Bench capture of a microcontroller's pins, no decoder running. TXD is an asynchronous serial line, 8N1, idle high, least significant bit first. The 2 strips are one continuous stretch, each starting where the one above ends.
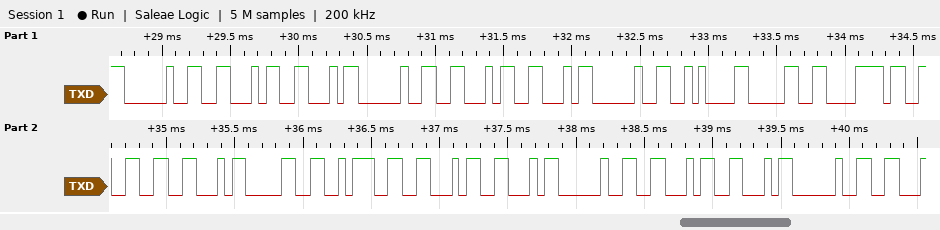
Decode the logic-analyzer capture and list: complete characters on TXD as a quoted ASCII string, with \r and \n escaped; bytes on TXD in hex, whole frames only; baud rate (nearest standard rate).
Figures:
" FF FF \n0x2F0:FF FF "
0x20 0x46 0x46 0x20 0x46 0x46 0x20 0x0A 0x30 0x78 0x32 0x46 0x30 0x3A 0x46 0x46 0x20 0x46 0x46 0x20
19200 baud
